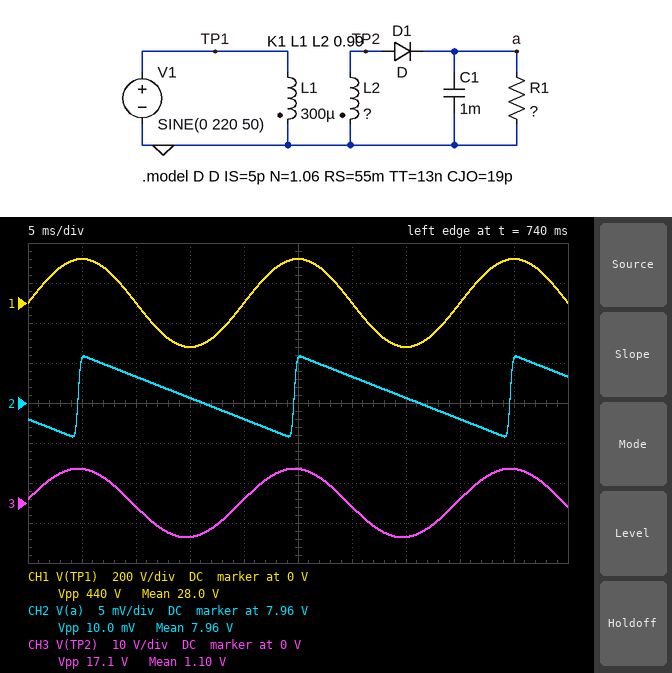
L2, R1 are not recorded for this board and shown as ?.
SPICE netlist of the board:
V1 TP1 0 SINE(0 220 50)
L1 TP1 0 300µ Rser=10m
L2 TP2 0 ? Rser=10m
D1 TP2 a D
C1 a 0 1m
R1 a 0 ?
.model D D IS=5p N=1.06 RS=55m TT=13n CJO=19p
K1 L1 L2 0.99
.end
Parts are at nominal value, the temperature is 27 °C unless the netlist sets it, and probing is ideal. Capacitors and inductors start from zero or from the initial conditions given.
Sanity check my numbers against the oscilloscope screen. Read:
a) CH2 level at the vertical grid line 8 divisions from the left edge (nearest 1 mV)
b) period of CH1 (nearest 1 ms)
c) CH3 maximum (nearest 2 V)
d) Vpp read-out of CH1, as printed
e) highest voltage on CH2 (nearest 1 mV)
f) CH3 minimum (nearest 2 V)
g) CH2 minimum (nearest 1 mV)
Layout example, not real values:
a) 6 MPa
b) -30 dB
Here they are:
a) 7.958 V
b) 20 ms
c) 8 V
d) 440 V
e) 7.966 V
f) -8 V
g) 7.956 V
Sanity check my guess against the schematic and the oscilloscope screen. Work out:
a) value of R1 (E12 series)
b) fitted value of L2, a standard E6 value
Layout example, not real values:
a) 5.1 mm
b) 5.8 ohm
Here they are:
a) 15 kΩ
b) 470 nH
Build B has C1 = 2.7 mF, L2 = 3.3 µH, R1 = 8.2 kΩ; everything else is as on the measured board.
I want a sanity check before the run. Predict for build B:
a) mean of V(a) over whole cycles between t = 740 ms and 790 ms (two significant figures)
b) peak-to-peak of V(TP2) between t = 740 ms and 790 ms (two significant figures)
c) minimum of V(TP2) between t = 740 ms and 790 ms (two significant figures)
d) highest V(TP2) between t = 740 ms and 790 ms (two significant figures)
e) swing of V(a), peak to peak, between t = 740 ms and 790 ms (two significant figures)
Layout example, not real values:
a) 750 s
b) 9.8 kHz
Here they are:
a) 22 V
b) 45 V
c) -23 V
d) 23 V
e) 19 mV
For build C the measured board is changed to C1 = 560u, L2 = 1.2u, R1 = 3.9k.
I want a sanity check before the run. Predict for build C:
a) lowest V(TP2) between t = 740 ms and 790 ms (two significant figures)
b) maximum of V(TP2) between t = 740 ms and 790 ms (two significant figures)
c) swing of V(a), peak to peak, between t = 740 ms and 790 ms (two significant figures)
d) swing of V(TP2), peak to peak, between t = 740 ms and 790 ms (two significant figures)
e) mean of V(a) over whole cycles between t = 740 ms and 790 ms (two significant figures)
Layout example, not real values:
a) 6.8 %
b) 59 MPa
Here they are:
a) -14 V
b) 14 V
c) 110 mV
d) 27 V
e) 13 V
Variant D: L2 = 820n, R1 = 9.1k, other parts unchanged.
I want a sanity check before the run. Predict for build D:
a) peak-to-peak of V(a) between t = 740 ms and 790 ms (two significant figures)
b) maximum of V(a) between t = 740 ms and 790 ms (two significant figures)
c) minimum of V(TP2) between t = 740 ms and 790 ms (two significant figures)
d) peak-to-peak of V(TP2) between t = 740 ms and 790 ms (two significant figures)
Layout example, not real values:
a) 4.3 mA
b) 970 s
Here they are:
a) 22 mV
b) 11 V
c) -11 V
d) 23 V
